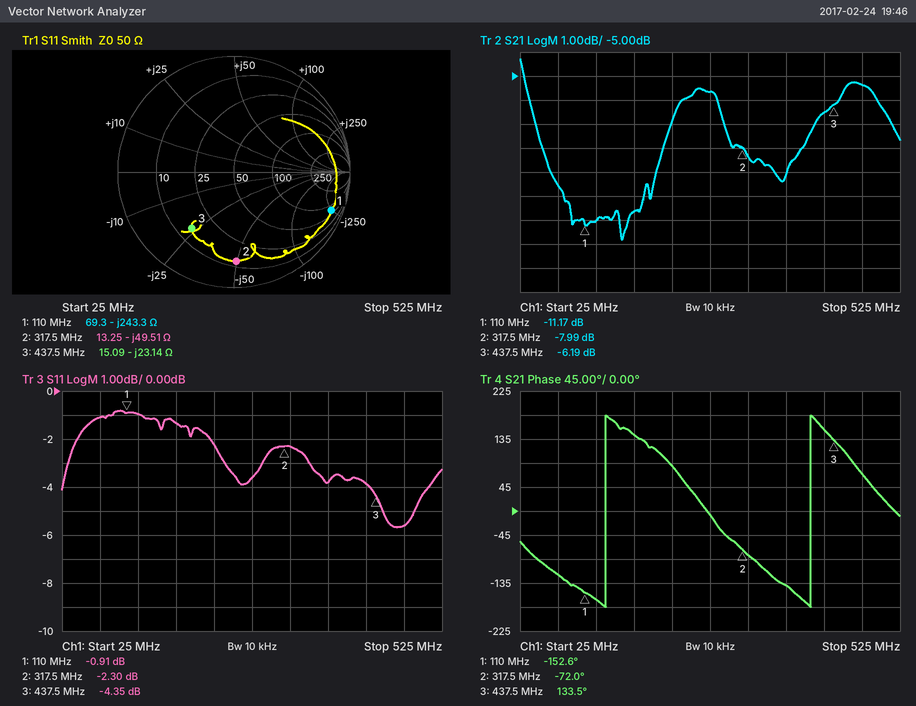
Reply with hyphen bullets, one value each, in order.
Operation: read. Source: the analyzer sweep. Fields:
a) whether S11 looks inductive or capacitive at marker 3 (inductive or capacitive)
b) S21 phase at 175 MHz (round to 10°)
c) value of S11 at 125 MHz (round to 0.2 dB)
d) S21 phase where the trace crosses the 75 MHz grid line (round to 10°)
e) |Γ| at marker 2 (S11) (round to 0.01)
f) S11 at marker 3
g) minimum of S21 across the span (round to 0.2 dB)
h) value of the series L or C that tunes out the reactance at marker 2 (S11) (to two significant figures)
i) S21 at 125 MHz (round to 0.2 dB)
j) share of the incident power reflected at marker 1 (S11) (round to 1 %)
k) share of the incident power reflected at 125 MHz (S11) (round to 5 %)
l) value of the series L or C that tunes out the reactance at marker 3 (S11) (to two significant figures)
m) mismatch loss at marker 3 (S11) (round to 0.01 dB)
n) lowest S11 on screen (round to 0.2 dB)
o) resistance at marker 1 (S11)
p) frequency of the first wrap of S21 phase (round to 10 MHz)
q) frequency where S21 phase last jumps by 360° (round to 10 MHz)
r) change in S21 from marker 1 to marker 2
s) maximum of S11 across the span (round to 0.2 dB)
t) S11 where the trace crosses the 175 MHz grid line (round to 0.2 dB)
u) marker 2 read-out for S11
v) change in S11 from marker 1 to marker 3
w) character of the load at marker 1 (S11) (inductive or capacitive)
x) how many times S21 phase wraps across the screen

- capacitive
- 140°
- -1.0 dB
- -120°
- 0.77
- -4.35 dB
- -11.8 dB
- 25 nH
- -11.0 dB
- 81 %
- 80 %
- 8.4 nH
- 1.99 dB
- -5.6 dB
- 69.3 Ω
- 140 MHz
- 410 MHz
- 3.18 dB
- -0.8 dB
- -1.4 dB
- -2.30 dB
- -3.44 dB
- capacitive
- 2
